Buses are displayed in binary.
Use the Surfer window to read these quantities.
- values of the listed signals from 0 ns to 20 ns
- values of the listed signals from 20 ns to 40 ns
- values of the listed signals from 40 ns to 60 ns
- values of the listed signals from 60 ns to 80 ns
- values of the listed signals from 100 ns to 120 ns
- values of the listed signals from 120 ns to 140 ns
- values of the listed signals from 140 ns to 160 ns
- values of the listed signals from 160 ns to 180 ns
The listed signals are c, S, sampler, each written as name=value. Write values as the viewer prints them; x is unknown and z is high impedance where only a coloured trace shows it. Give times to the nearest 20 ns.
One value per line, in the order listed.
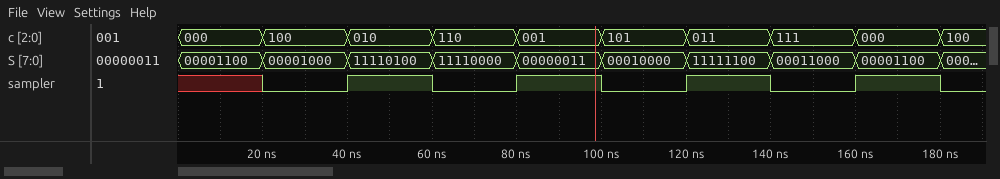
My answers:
c=000, S=00001100, sampler=x
c=100, S=00001000, sampler=0
c=010, S=11110100, sampler=1
c=110, S=11110000, sampler=0
c=101, S=00010000, sampler=0
c=011, S=11111100, sampler=1
c=111, S=00011000, sampler=0
c=000, S=00001100, sampler=1
